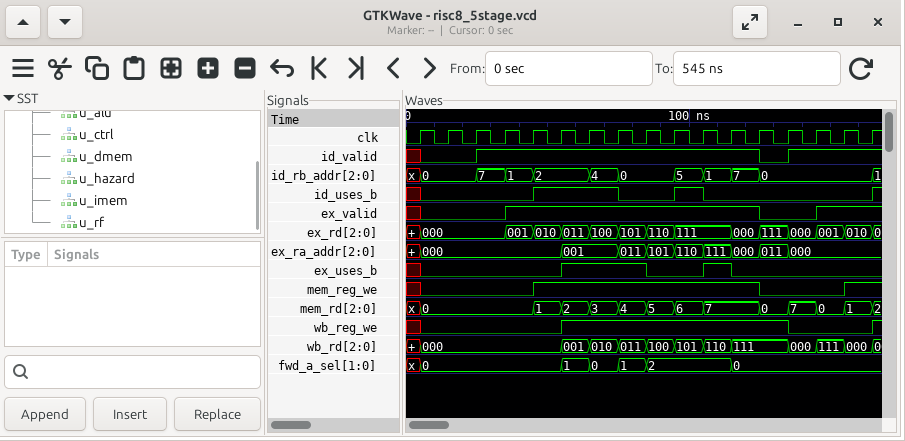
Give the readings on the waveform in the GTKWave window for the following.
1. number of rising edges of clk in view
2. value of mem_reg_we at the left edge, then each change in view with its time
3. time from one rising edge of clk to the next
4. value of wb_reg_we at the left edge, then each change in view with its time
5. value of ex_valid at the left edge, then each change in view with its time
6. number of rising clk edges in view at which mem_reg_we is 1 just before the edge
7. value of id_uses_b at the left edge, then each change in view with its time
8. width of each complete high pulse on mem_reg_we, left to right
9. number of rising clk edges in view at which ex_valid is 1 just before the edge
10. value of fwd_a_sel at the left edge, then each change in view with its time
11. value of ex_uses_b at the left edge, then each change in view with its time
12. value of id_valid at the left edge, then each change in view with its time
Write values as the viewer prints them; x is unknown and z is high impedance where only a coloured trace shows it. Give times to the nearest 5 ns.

17
x, 0 at 5 ns, 1 at 45 ns, 0 at 125 ns, 1 at 155 ns
10 ns
x, 0 at 5 ns, 1 at 55 ns, 0 at 135 ns, 1 at 165 ns
x, 0 at 5 ns, 1 at 35 ns, 0 at 125 ns, 1 at 145 ns
9
x, 0 at 5 ns, 1 at 45 ns, 0 at 75 ns, 1 at 95 ns, 0 at 105 ns, 1 at 165 ns
80 ns
11
x, 0 at 5 ns, 1 at 55 ns, 0 at 65 ns, 1 at 75 ns, 2 at 85 ns, 0 at 115 ns
x, 0 at 5 ns, 1 at 55 ns, 0 at 85 ns, 1 at 105 ns, 0 at 115 ns
x, 0 at 5 ns, 1 at 25 ns, 0 at 125 ns, 1 at 135 ns
